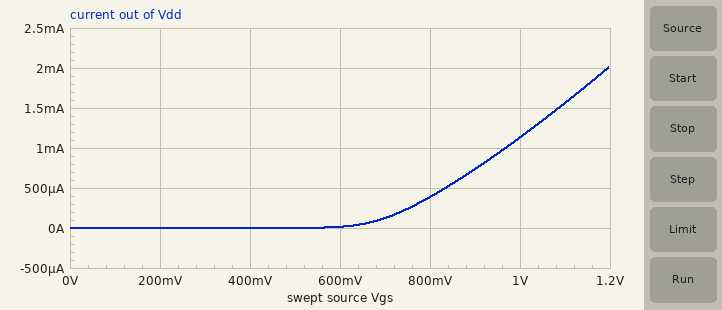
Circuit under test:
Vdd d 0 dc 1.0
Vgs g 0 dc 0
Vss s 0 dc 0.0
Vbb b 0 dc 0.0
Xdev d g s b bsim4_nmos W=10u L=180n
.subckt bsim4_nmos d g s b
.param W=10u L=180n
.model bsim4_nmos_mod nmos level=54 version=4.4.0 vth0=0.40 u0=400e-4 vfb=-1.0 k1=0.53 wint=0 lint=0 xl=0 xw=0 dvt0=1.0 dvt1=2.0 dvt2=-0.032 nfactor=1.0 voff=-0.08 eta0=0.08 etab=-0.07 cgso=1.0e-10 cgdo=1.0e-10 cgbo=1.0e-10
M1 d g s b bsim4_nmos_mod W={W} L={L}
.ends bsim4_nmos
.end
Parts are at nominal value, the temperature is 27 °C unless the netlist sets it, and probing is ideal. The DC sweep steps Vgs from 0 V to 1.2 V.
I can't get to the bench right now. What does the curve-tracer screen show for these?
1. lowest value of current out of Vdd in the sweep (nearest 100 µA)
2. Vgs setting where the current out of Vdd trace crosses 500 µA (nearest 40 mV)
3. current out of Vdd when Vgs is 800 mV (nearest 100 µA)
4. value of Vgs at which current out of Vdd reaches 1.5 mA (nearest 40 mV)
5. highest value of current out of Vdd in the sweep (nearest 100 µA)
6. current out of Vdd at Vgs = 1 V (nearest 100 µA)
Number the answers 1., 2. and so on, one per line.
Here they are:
1. 0 A
2. 840 mV
3. 400 µA
4. 1.08 V
5. 2.0 mA
6. 1.1 mA
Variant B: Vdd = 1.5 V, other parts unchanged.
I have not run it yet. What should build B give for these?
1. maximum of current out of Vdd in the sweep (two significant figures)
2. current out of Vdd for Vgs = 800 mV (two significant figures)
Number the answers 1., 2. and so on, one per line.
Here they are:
1. 2.2 mA
2. 440 µA
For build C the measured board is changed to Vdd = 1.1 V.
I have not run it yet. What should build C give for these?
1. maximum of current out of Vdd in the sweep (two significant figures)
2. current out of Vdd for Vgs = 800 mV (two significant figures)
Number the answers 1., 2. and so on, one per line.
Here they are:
1. 2.1 mA
2. 400 µA
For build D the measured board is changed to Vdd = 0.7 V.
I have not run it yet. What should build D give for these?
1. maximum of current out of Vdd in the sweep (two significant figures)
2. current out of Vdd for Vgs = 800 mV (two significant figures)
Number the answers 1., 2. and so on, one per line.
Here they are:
1. 1.9 mA
2. 350 µA
